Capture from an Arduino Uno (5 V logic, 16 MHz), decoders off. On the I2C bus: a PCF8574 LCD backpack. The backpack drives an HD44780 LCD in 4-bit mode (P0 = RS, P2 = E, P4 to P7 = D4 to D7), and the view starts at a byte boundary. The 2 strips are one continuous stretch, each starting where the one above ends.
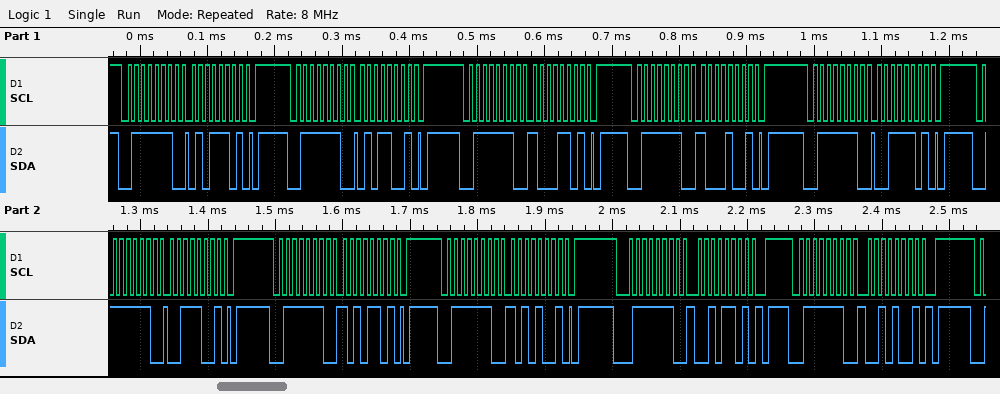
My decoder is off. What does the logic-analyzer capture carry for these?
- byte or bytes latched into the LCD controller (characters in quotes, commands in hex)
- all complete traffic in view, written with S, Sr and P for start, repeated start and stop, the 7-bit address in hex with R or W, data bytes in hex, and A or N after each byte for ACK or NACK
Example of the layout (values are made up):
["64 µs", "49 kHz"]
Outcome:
["'X' ':'", "S 3FW A 5D A P S 3FW A 59 A P S 3FW A 8D A P S 3FW A 89 A P S 3FW A 3D A P S 3FW A 39 A P S 3FW A AD A P S 3FW A A9 A P S 3FW A 2D A P S 3FW A 29 A P"]
